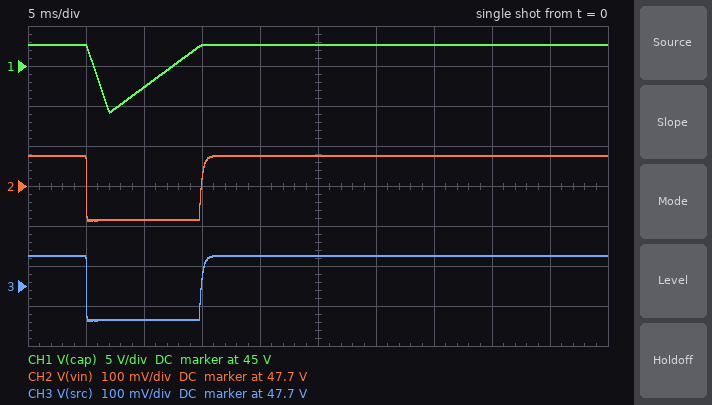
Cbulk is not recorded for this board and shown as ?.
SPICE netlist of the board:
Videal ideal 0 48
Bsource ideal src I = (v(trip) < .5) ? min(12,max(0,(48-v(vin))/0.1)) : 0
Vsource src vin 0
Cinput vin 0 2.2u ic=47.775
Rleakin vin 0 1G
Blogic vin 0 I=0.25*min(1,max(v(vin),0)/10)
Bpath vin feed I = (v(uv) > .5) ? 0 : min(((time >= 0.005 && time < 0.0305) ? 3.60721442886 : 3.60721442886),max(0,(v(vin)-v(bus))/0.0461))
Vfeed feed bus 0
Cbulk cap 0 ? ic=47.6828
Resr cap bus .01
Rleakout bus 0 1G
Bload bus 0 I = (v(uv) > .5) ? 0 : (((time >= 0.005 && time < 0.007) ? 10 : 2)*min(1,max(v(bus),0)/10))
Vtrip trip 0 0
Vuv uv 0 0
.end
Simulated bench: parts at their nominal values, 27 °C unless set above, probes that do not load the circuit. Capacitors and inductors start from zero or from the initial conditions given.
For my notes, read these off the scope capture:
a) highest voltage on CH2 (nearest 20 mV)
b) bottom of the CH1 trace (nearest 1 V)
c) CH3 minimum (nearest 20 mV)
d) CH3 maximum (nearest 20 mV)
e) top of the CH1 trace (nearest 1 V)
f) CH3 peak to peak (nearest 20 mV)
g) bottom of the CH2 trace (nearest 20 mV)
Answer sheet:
47.78 V
39 V
47.62 V
47.78 V
48 V
160 mV
47.62 V
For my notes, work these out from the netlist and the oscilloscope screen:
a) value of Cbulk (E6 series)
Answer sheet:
1.5 mF
